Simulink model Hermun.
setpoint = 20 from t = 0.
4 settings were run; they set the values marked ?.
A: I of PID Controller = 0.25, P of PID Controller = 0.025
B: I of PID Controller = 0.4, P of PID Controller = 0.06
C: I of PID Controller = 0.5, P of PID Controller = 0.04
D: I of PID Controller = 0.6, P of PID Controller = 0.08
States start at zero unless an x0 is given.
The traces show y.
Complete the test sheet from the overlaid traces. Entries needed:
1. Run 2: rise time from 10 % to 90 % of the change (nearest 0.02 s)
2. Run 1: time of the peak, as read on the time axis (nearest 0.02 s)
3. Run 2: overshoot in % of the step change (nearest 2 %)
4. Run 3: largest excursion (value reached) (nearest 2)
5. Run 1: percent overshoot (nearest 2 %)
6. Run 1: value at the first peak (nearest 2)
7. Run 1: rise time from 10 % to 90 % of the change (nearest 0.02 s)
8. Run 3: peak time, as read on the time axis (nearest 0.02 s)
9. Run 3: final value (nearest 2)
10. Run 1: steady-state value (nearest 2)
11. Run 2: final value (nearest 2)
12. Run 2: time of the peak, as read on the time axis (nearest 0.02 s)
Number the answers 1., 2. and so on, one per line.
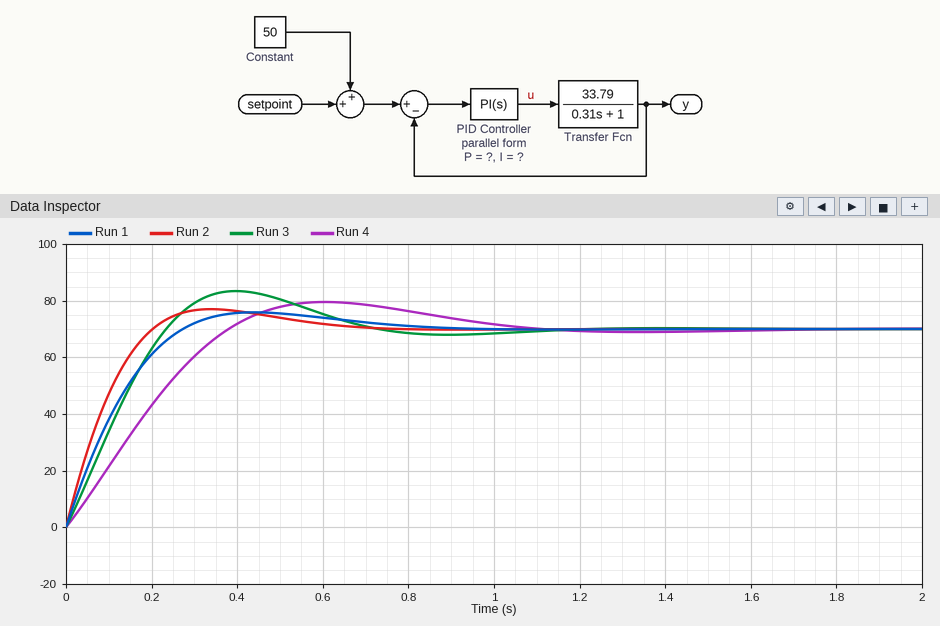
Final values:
1. 0.14 s
2. 0.44 s
3. 10 %
4. 84
5. 8 %
6. 76
7. 0.20 s
8. 0.40 s
9. 70
10. 70
11. 70
12. 0.34 s
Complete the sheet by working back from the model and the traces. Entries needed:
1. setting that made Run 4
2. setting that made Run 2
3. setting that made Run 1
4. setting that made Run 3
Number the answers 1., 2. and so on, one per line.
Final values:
1. A
2. D
3. B
4. C
